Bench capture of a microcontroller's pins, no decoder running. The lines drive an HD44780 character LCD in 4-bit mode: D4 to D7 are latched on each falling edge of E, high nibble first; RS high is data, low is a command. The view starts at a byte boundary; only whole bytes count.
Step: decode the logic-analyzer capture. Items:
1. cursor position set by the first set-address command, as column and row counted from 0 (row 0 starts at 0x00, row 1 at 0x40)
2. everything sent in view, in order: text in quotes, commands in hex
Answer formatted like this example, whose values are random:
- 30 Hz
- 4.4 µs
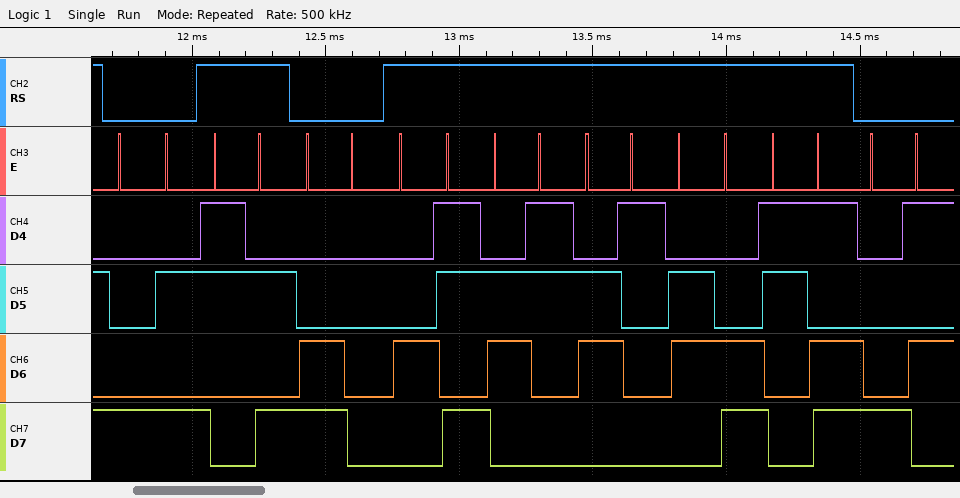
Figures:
- column 10, row 0
- 0x8A ":" 0xC0 "Kcal=" 0x85
